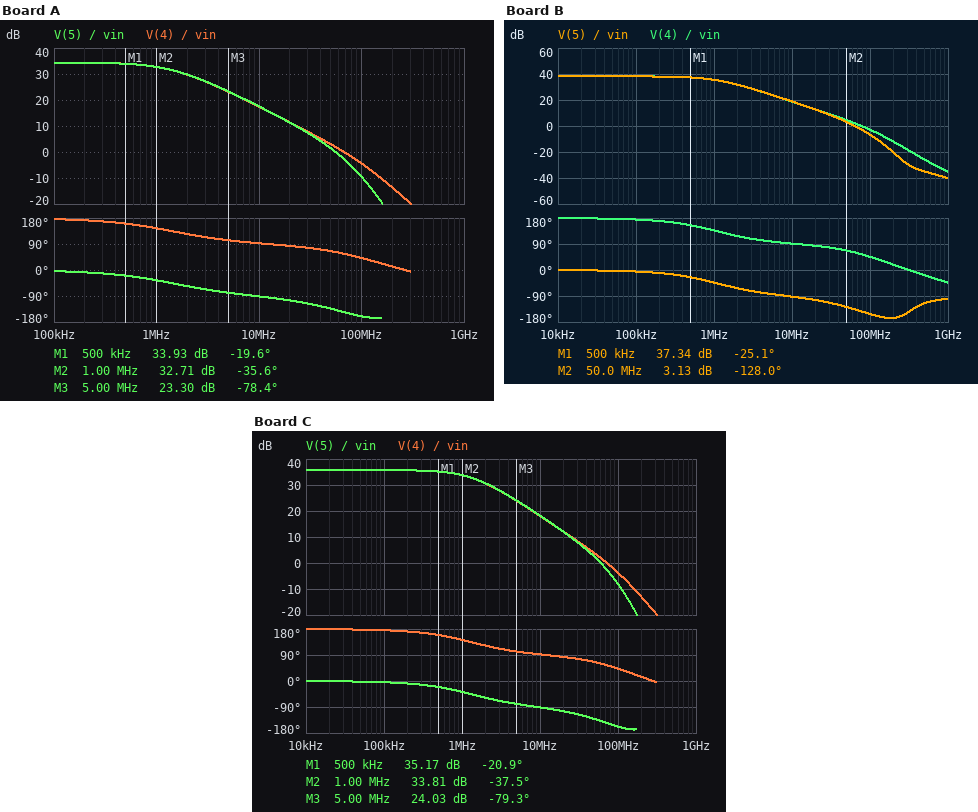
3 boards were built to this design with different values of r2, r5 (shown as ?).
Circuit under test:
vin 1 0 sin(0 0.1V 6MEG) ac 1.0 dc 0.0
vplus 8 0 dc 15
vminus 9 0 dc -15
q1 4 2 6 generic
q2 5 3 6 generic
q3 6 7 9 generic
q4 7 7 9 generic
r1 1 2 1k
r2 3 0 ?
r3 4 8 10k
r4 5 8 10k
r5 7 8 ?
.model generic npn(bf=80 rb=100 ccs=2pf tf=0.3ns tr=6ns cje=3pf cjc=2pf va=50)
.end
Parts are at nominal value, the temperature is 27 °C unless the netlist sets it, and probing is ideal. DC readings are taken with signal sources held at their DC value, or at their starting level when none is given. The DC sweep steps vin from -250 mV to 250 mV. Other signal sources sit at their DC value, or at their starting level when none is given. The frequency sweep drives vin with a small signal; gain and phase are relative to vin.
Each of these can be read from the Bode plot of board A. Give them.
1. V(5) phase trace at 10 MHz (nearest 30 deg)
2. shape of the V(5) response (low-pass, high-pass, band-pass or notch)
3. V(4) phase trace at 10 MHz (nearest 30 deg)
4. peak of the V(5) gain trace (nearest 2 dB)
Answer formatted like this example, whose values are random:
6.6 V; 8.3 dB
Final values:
-90 deg; low-pass; 90 deg; 34 dB
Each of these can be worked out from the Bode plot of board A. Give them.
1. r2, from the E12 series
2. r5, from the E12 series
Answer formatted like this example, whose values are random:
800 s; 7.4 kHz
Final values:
680 Ω; 56 kΩ
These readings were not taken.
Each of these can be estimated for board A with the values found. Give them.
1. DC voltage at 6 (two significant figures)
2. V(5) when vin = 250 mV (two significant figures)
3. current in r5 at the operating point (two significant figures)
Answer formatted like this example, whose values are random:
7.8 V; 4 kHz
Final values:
-740 mV; 15 V; 520 µA
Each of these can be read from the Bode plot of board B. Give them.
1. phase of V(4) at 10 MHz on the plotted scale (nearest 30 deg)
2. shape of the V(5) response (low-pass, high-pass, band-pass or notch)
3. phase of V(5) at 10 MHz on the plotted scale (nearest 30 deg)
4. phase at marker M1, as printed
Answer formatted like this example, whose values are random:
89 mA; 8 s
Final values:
90 deg; low-pass; -90 deg; -25.1 deg
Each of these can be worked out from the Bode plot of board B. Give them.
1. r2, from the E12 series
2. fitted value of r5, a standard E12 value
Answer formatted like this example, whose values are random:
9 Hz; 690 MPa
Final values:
470 Ω; 33 kΩ
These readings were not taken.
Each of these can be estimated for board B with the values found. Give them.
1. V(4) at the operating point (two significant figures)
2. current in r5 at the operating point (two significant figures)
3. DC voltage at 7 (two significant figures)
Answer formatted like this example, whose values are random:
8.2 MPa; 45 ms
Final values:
9.8 V; 890 µA; -14 V
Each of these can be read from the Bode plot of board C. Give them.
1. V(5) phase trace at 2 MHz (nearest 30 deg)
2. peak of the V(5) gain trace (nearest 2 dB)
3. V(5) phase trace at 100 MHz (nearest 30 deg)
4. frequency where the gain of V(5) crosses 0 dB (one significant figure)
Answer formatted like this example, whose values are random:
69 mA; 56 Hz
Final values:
-60 deg; 36 dB; -150 deg; 60 MHz
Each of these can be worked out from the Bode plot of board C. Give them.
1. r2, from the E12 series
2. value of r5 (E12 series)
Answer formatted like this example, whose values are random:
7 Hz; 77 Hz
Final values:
560 Ω; 47 kΩ
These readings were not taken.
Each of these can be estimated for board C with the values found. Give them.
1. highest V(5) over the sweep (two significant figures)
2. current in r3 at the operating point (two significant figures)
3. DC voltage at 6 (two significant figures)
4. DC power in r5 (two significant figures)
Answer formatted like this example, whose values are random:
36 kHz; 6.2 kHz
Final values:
15 V; 370 µA; -750 mV; 18 mW
